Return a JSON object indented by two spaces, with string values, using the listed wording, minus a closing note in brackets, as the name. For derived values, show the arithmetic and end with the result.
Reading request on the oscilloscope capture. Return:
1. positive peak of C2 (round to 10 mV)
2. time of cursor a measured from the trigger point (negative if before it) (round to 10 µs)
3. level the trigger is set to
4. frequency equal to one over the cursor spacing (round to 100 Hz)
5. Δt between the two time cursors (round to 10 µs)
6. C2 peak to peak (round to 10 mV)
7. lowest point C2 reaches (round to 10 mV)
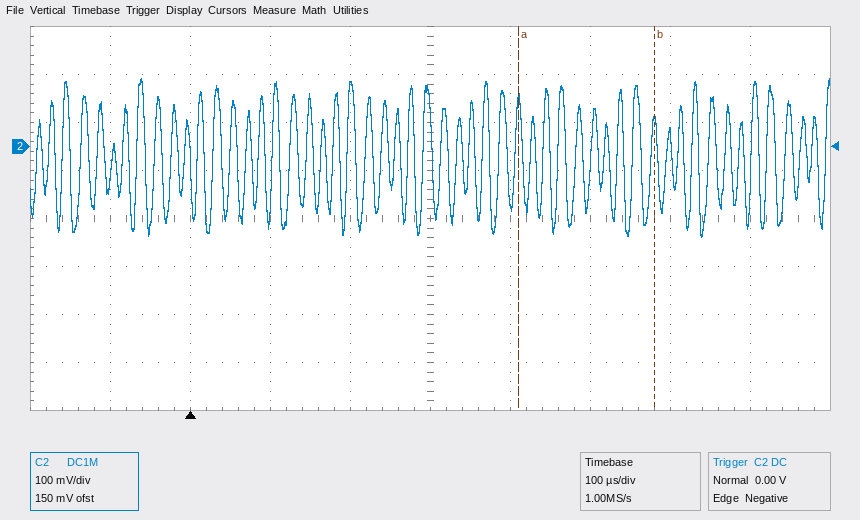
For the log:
{
  "positive peak of C2": "140 mV",
  "time of cursor a measured from the trigger point (negative if before it)": "+410 µs",
  "level the trigger is set to": "0.00 V",
  "frequency equal to one over the cursor spacing": "1 / 170 µs ≈ 5.9 kHz",
  "Δt between the two time cursors": "170 µs",
  "C2 peak to peak": "140 mV − (-190 mV) = 330 mV",
  "lowest point C2 reaches": "-190 mV"
}
